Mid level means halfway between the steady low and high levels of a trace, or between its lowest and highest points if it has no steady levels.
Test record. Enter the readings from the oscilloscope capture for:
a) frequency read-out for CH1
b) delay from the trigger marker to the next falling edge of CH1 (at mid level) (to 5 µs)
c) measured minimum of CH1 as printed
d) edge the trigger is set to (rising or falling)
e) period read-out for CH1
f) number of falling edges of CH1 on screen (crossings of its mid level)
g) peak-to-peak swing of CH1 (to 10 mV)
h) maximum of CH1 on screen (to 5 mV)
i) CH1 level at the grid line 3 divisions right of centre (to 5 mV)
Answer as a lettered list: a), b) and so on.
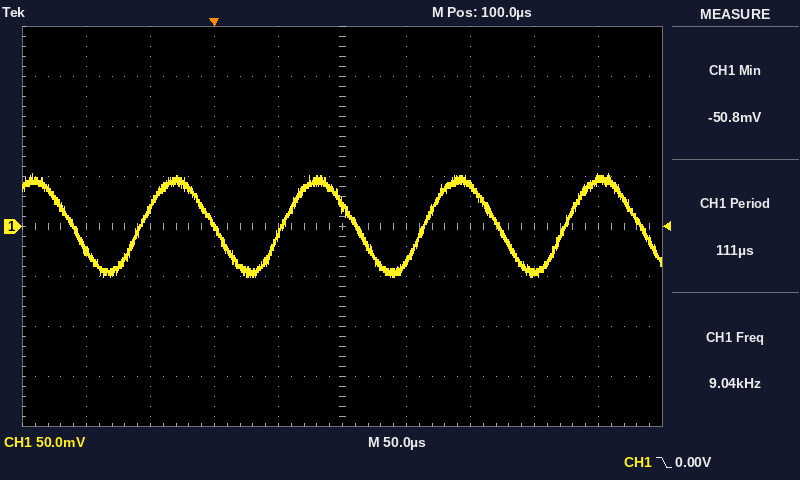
a) 9.04 kHz
b) 110 µs
c) -50.8 mV
d) falling
e) 111 µs
f) 5
g) 100 mV
h) 55 mV
i) -45 mV
